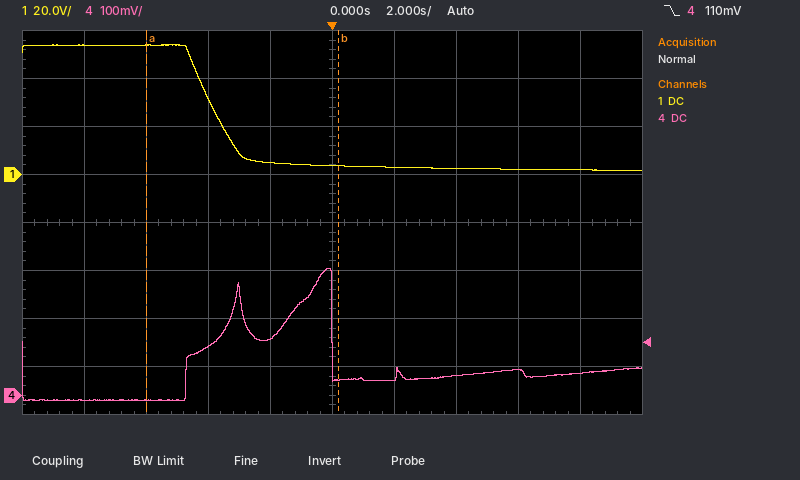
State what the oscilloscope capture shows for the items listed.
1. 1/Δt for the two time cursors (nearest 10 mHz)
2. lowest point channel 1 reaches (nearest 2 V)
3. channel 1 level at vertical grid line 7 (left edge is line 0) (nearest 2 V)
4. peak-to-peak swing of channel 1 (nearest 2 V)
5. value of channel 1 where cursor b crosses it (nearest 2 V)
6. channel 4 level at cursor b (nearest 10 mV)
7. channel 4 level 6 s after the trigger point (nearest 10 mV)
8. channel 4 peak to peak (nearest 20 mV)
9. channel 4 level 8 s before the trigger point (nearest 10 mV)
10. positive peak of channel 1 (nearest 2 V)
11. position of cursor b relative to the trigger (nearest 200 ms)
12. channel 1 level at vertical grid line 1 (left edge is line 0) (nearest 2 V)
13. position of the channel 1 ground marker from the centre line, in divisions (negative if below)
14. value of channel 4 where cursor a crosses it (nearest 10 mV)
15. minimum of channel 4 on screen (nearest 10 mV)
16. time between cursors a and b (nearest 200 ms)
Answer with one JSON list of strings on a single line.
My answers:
["160 mHz", "2 V", "2 V", "52 V", "4 V", "30 mV", "50 mV", "280 mV", "-10 mV", "54 V", "+200 ms", "54 V", "+1.0 div", "-10 mV", "-10 mV", "6.2 s"]
